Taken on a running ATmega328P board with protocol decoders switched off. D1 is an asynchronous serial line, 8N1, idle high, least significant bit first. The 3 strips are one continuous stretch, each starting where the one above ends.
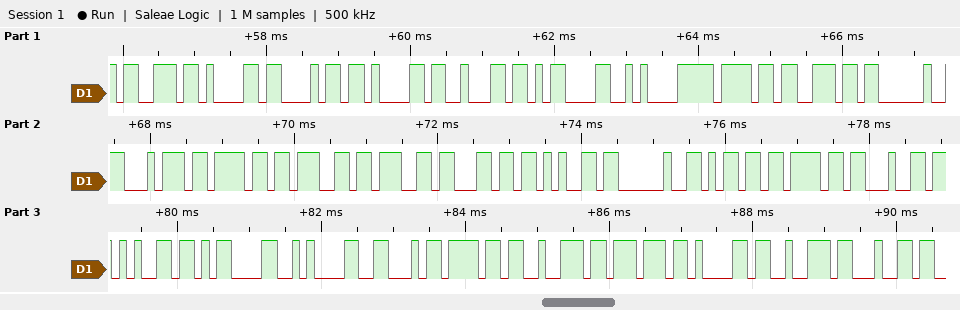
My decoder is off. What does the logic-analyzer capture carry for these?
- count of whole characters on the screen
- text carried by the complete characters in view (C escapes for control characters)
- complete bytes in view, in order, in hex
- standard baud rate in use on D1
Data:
30
"sahab\r\non toggle mode\r\nForward"
73 61 68 61 62 0D 0A 6F 6E 20 74 6F 67 67 6C 65 20 6D 6F 64 65 0D 0A 46 6F 72 77 61 72 64
9600 baud
